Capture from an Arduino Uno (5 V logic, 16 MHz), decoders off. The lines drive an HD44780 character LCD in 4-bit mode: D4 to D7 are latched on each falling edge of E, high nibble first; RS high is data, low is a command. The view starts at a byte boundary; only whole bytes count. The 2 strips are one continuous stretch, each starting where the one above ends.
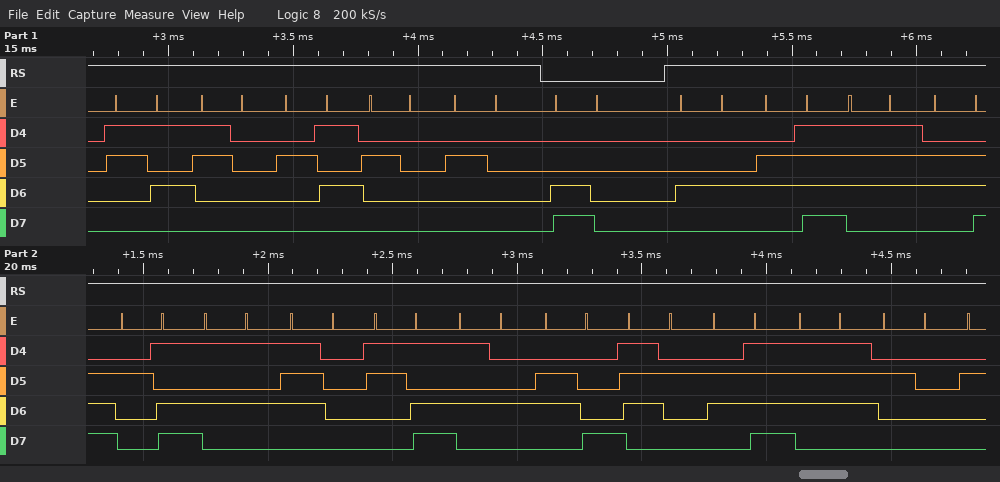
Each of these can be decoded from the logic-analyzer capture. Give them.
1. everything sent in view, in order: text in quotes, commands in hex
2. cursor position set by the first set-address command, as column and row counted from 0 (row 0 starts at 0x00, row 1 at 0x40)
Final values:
"50%  " 0xC0 "Down-Up=Throw "
column 0, row 1
